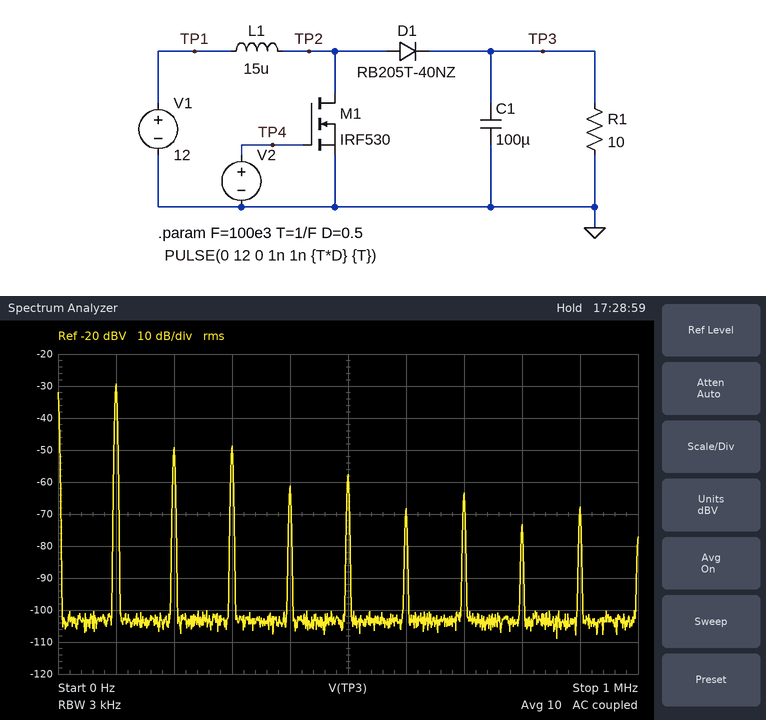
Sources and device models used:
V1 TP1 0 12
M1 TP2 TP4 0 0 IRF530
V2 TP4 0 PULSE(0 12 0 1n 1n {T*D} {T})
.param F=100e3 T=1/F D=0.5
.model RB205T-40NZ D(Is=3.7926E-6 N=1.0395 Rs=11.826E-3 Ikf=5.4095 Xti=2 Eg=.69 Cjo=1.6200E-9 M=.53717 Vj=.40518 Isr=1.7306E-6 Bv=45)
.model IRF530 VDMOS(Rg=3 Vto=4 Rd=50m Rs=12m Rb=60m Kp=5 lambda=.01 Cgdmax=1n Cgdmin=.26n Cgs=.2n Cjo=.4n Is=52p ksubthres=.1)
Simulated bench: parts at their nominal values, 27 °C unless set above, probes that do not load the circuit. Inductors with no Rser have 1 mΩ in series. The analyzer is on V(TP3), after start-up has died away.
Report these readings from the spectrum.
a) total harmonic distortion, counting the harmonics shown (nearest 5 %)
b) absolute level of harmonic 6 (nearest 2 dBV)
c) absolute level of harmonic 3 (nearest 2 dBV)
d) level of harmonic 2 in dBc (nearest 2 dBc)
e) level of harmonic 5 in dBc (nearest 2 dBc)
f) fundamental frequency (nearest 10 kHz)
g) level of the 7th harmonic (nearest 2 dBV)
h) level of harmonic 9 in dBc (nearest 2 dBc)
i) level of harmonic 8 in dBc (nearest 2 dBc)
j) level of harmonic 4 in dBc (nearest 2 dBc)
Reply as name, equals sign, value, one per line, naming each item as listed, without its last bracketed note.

total harmonic distortion, counting the harmonics shown = 15 %
absolute level of harmonic 6 = -68 dBV
absolute level of harmonic 3 = -48 dBV
level of harmonic 2 in dBc = -20 dBc
level of harmonic 5 in dBc = -28 dBc
fundamental frequency = 100 kHz
level of the 7th harmonic = -64 dBV
level of harmonic 9 in dBc = -38 dBc
level of harmonic 8 in dBc = -44 dBc
level of harmonic 4 in dBc = -32 dBc
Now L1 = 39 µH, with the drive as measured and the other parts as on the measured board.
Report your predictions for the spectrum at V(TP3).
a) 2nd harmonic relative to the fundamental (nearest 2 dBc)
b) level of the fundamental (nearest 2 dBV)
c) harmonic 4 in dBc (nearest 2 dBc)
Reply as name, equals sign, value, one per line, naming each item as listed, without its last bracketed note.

2nd harmonic relative to the fundamental = -28 dBc
level of the fundamental = -30 dBV
harmonic 4 in dBc = -40 dBc
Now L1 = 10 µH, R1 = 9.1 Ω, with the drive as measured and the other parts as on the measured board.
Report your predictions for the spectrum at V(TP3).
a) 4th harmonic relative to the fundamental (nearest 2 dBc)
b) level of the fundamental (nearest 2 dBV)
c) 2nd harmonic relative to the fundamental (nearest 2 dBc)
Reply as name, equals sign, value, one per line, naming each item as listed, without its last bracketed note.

4th harmonic relative to the fundamental = -30 dBc
level of the fundamental = -28 dBV
2nd harmonic relative to the fundamental = -18 dBc
